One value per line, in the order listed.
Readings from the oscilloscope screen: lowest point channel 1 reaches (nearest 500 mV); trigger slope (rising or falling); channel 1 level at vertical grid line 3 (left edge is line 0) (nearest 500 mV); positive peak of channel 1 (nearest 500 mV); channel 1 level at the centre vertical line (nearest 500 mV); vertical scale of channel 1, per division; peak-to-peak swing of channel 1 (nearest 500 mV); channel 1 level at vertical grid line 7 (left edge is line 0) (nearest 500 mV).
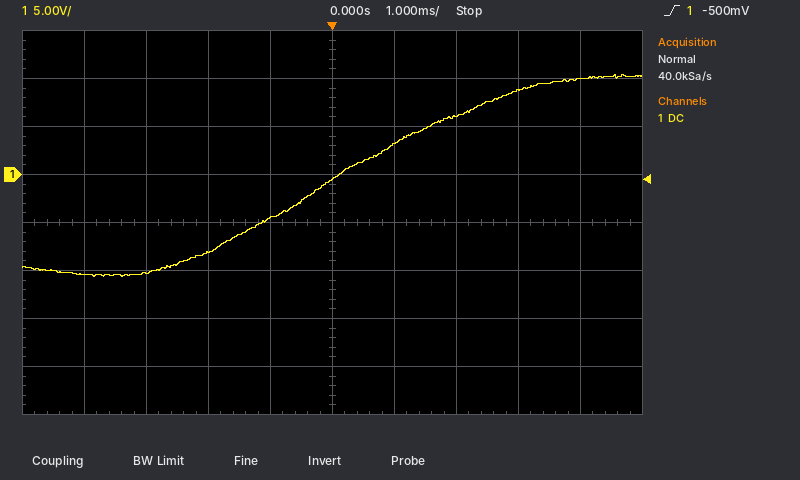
-10.5 V
rising
-8.0 V
10.5 V
-500 mV
5 V
21.0 V
6.0 V
